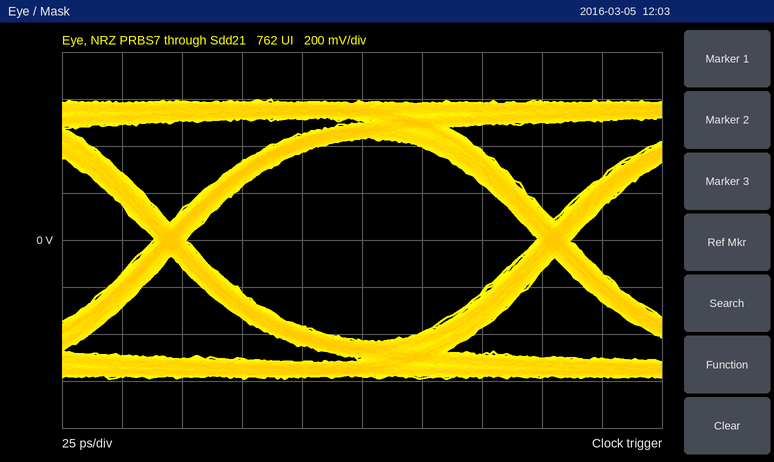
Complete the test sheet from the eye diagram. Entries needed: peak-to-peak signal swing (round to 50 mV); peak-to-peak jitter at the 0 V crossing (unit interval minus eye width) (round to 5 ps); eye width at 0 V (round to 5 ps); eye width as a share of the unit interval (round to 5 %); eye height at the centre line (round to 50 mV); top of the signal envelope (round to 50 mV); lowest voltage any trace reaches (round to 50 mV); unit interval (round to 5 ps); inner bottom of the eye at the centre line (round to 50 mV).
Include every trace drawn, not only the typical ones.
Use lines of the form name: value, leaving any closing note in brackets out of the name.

peak-to-peak signal swing: 1.20 V
peak-to-peak jitter at the 0 V crossing (unit interval minus eye width): 15 ps
eye width at 0 V: 145 ps
eye width as a share of the unit interval: 90 %
eye height at the centre line: 850 mV
top of the signal envelope: 600 mV
lowest voltage any trace reaches: -600 mV
unit interval: 160 ps
inner bottom of the eye at the centre line: -450 mV
